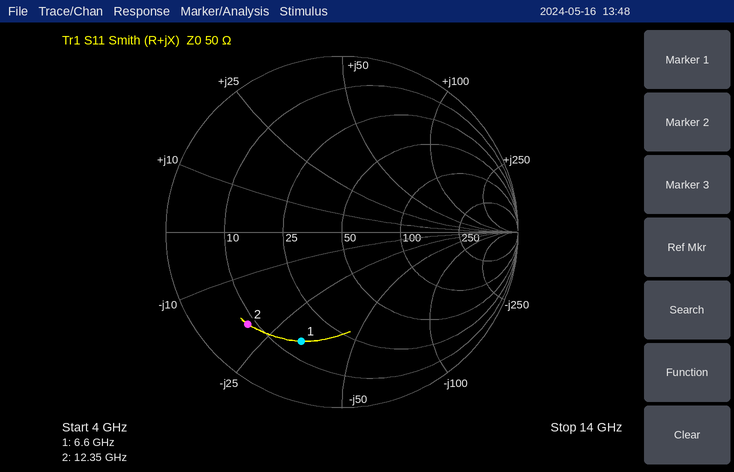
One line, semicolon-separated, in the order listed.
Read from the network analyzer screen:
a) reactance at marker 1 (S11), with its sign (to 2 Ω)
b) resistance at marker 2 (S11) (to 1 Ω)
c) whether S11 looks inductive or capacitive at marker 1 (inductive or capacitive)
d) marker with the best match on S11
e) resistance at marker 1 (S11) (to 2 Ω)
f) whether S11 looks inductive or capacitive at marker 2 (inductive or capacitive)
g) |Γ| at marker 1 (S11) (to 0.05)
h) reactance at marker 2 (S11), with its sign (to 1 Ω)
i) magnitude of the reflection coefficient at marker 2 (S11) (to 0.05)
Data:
-32 Ω; 8 Ω; capacitive; marker 1; 14 Ω; capacitive; 0.65; -20 Ω; 0.75
